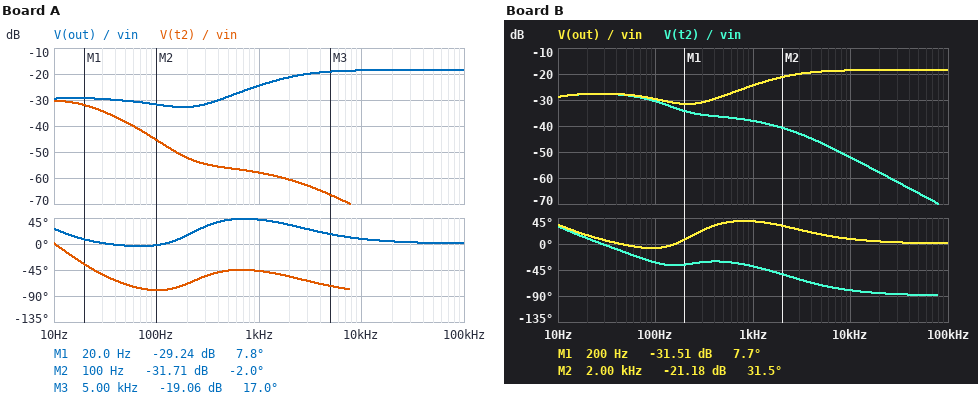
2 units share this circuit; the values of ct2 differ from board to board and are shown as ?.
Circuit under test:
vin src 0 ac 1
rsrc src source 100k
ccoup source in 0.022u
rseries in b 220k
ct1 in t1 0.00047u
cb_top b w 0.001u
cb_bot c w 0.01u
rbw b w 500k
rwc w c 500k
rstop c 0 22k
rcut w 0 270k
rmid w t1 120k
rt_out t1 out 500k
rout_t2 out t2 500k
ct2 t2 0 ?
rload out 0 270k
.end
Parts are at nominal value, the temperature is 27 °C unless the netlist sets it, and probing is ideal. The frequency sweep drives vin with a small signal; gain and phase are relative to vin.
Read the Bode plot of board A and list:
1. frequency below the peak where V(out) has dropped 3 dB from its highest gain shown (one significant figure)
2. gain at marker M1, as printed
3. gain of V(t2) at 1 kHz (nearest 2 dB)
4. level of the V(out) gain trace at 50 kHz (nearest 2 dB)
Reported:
2 kHz
-29.24 dB
-58 dB
-18 dB
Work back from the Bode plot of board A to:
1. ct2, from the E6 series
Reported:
15 nF
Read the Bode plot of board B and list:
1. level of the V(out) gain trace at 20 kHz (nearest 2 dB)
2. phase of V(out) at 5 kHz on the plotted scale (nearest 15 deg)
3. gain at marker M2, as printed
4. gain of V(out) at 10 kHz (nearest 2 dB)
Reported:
-18 dB
15 deg
-21.18 dB
-18 dB
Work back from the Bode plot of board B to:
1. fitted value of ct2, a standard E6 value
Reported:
1.5 nF
